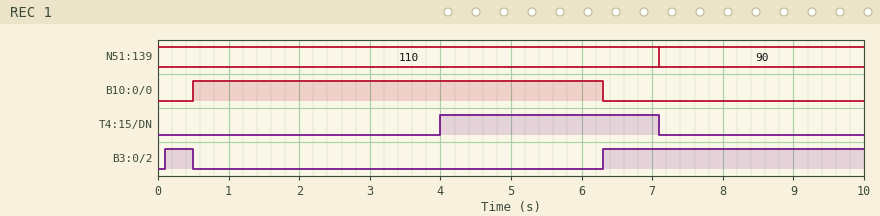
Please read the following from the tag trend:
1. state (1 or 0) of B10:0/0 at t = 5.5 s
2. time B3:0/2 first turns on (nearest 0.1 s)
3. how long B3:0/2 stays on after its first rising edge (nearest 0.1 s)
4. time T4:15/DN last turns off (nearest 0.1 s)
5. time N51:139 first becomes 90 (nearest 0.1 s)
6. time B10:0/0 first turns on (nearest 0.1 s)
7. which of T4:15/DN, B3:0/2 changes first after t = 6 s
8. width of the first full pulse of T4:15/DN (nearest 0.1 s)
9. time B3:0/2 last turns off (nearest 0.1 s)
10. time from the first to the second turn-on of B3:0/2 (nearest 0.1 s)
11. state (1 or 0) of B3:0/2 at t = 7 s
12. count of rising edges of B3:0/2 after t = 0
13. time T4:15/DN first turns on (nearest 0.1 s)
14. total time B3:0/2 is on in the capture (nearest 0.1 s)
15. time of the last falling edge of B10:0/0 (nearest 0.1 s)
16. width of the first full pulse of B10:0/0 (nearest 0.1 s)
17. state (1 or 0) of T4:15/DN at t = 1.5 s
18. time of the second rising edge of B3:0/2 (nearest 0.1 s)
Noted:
1
0.1 s
0.4 s
7.1 s
7.1 s
0.5 s
B3:0/2
3.1 s
0.5 s
6.2 s
1
2
4.0 s
4.1 s
6.3 s
5.8 s
0
6.3 s
